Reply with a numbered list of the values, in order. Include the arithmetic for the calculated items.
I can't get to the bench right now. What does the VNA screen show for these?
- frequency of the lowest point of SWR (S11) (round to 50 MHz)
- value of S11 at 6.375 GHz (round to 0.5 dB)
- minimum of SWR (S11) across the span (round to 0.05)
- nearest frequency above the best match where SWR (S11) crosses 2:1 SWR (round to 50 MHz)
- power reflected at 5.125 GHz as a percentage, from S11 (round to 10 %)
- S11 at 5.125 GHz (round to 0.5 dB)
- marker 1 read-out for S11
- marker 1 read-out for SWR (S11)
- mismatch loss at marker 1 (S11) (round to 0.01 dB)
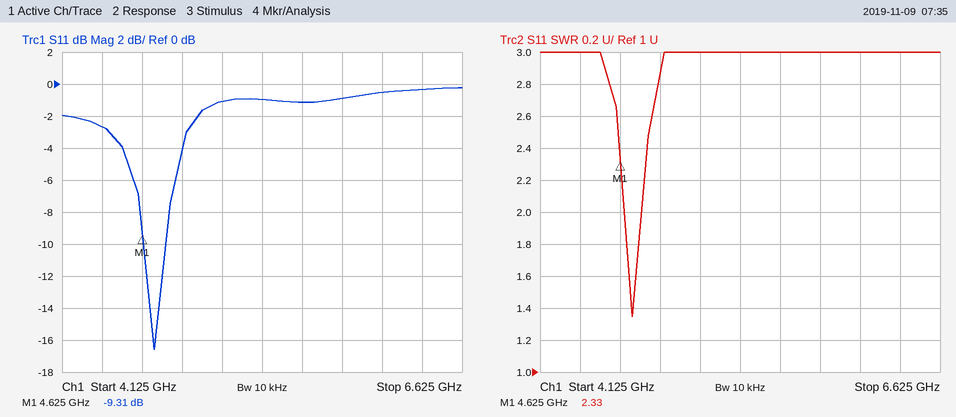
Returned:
1. 4.70 GHz
2. -0.5 dB
3. 1.35
4. 4.75 GHz
5. 10^(-1/10) ≈ 79.4 %, so 80 % to the nearest 10 %
6. -1.0 dB
7. -9.31 dB
8. 2.33
9. −10 log10(1 − 10^(-9.31/10)) ≈ 0.54 dB
